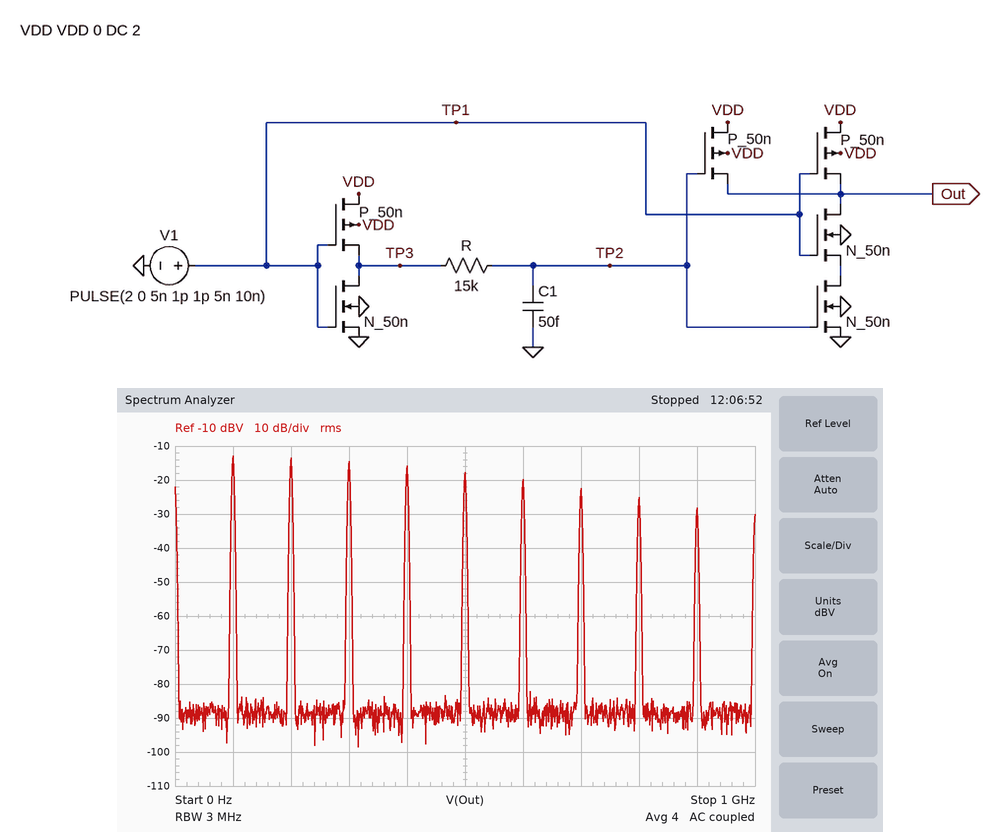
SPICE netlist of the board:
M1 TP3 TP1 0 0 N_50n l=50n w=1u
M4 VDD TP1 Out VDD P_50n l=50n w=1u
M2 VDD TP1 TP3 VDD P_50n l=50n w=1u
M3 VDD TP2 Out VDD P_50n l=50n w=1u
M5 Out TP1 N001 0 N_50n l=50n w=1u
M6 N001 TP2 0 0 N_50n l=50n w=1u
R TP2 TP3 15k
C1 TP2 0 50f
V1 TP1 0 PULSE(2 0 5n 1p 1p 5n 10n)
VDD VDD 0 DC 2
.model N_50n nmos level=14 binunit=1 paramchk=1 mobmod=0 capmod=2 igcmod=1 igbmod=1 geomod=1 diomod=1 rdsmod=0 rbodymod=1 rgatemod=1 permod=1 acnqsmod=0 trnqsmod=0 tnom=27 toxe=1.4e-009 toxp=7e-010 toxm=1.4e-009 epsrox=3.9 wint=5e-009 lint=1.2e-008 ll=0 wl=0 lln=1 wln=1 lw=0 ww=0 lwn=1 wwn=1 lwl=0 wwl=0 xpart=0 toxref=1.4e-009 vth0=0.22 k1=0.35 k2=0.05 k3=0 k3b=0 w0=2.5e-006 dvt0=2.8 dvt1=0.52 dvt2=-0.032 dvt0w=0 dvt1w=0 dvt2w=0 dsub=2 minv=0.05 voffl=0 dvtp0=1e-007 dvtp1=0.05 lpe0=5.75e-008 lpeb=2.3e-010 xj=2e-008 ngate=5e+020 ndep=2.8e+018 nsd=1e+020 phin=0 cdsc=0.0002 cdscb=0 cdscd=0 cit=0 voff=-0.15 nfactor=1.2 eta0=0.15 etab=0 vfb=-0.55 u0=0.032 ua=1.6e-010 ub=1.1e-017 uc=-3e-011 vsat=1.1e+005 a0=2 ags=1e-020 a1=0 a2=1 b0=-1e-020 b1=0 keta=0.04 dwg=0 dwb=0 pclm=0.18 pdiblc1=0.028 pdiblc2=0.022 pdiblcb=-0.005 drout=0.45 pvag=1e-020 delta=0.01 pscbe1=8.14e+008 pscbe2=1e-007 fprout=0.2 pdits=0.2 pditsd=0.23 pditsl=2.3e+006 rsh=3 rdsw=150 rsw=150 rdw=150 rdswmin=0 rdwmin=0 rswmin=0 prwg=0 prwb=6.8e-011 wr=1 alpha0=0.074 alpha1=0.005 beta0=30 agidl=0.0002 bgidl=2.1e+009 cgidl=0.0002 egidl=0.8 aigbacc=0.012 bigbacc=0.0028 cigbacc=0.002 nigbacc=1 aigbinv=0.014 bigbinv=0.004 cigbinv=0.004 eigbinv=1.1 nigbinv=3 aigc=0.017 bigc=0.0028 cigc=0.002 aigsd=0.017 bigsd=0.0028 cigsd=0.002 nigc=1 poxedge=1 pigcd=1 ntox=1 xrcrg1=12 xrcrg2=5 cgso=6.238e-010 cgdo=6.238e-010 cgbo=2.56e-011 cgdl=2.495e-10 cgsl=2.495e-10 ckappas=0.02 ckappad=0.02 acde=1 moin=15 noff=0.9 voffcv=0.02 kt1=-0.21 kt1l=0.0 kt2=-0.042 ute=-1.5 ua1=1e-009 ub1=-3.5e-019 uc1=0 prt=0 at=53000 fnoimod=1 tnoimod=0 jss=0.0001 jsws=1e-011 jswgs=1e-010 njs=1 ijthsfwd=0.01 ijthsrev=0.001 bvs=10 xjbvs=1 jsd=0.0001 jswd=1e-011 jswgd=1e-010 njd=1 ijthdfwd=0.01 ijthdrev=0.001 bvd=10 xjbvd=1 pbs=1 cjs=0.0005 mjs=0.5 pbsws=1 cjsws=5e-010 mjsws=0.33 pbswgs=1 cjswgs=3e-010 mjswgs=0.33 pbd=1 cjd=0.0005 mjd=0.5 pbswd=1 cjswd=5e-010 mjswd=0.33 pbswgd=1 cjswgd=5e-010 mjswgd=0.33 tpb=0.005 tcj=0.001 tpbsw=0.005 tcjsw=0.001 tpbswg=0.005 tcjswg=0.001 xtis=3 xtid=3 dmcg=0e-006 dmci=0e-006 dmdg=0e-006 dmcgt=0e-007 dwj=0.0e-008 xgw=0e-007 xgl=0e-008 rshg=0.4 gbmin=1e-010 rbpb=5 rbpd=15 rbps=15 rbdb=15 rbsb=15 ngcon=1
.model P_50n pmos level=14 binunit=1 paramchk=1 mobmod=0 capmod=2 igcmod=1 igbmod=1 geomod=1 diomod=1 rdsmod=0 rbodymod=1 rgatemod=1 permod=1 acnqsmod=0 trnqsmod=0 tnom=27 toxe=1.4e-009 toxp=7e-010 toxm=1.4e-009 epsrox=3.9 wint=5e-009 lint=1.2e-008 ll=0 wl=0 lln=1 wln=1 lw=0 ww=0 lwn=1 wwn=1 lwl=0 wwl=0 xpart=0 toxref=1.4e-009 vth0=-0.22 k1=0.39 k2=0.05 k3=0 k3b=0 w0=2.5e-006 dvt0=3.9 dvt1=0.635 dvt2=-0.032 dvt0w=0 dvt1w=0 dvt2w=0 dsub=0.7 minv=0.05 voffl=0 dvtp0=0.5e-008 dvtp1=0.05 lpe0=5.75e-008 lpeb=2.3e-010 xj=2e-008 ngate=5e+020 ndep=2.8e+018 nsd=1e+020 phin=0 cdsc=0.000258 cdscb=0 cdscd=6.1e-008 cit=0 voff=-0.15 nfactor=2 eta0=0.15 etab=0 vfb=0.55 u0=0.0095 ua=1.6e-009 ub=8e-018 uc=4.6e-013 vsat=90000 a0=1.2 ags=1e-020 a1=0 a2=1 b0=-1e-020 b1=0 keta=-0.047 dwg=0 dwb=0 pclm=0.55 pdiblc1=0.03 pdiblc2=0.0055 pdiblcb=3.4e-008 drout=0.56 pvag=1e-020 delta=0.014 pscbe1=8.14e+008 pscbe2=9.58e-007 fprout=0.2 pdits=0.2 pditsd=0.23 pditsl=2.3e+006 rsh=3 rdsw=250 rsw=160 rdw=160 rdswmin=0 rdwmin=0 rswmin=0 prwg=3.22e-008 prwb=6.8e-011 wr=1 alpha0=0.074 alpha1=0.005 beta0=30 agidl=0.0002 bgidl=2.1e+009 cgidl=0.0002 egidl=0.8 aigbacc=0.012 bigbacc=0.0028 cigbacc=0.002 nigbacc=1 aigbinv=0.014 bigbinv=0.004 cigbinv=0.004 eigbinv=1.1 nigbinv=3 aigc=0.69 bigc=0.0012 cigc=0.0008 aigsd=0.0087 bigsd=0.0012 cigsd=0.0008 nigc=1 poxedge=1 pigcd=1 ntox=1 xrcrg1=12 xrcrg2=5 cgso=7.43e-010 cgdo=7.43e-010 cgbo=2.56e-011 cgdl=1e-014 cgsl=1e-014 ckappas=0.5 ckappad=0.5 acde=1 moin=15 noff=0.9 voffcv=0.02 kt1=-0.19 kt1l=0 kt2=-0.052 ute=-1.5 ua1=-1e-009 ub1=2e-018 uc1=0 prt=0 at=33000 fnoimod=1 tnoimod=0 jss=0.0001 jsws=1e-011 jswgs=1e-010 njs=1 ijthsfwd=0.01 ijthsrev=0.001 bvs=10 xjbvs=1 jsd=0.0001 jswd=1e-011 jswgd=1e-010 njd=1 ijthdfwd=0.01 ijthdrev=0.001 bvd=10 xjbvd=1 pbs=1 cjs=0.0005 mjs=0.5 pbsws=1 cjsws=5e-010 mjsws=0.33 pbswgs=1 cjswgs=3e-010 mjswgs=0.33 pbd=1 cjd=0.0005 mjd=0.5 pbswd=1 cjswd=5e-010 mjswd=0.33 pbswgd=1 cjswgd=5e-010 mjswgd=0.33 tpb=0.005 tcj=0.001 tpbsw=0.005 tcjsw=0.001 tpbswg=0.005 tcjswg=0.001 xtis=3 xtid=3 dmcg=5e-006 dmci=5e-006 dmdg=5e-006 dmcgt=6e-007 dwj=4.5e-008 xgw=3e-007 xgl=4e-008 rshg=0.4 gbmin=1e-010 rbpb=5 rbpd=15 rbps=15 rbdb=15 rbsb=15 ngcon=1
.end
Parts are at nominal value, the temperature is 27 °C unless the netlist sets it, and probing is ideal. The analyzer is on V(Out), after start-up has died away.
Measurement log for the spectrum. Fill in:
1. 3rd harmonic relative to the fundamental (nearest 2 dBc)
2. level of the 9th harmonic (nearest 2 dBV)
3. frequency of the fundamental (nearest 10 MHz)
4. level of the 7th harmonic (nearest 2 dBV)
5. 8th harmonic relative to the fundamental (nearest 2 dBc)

-2 dBc
-28 dBV
100 MHz
-22 dBV
-12 dBc
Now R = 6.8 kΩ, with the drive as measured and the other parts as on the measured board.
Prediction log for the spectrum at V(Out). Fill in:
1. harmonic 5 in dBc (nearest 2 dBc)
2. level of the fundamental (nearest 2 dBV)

-2 dBc
-18 dBV
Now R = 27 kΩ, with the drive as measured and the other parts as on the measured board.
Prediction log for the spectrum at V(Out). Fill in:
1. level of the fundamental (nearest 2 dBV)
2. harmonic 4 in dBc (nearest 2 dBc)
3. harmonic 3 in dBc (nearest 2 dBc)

-8 dBV
-8 dBc
-4 dBc
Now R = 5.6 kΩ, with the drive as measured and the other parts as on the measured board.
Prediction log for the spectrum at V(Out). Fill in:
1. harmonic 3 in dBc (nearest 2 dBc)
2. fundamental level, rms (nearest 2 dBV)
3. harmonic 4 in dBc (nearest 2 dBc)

0 dBc
-20 dBV
0 dBc
